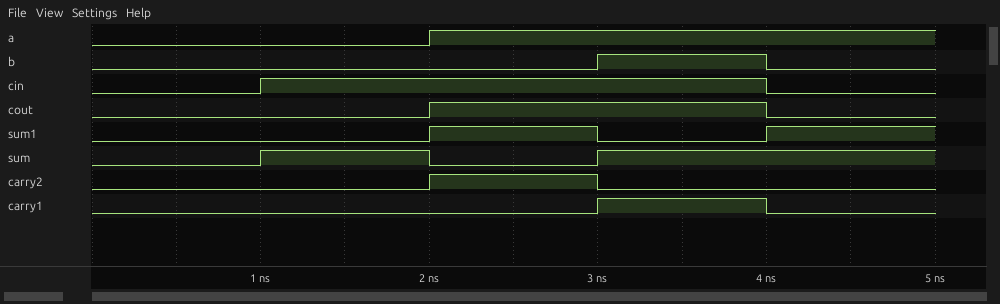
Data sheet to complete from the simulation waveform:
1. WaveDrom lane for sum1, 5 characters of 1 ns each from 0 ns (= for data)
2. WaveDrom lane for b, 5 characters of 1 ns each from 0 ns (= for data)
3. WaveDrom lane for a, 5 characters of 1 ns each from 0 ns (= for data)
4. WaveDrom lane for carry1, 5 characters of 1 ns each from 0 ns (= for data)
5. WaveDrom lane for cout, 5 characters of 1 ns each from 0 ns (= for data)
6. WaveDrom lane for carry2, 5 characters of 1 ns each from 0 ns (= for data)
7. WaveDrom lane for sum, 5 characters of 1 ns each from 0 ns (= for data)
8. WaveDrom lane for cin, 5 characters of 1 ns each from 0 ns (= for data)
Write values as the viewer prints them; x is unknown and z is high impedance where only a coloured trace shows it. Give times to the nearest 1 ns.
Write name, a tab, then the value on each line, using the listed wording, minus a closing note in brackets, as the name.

WaveDrom lane for sum1, 5 characters of 1 ns each from 0 ns	{name: 'sum1', wave: '0.101'}
WaveDrom lane for b, 5 characters of 1 ns each from 0 ns	{name: 'b', wave: '0..10'}
WaveDrom lane for a, 5 characters of 1 ns each from 0 ns	{name: 'a', wave: '0.1..'}
WaveDrom lane for carry1, 5 characters of 1 ns each from 0 ns	{name: 'carry1', wave: '0..10'}
WaveDrom lane for cout, 5 characters of 1 ns each from 0 ns	{name: 'cout', wave: '0.1.0'}
WaveDrom lane for carry2, 5 characters of 1 ns each from 0 ns	{name: 'carry2', wave: '0.10.'}
WaveDrom lane for sum, 5 characters of 1 ns each from 0 ns	{name: 'sum', wave: '0101.'}
WaveDrom lane for cin, 5 characters of 1 ns each from 0 ns	{name: 'cin', wave: '01..0'}
